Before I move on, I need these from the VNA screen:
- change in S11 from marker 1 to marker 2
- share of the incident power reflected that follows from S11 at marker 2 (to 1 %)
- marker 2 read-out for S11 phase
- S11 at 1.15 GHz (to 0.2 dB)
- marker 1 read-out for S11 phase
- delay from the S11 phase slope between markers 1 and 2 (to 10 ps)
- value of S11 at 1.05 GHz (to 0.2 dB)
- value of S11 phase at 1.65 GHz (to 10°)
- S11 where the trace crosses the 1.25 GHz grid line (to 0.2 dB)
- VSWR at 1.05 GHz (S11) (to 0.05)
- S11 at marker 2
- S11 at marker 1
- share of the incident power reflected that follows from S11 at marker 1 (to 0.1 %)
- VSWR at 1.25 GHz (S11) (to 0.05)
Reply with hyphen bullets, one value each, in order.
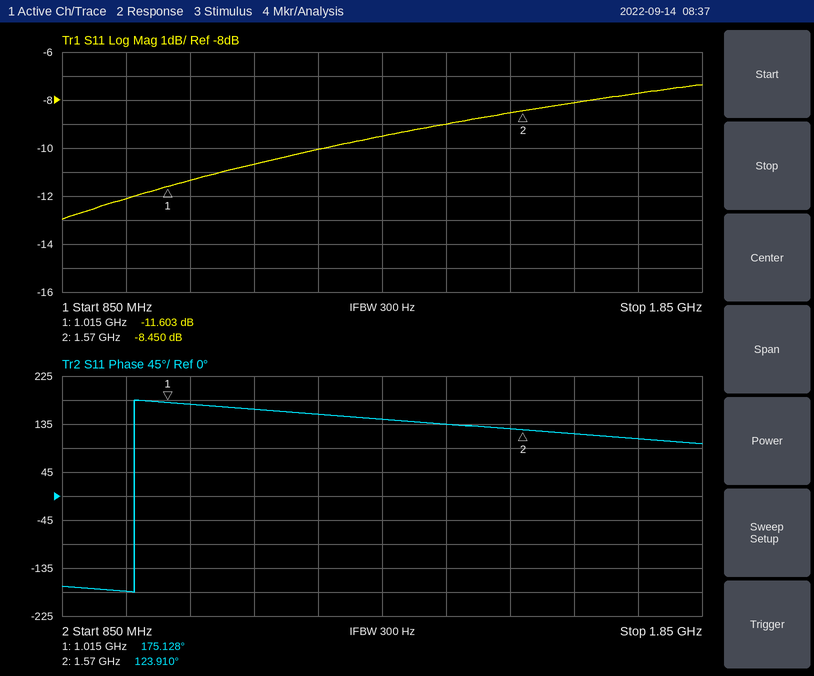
- 3.153 dB
- 14 %
- 123.910°
- -10.6 dB
- 175.128°
- 260 ps
- -11.4 dB
- 120°
- -10.0 dB
- 1.75
- -8.450 dB
- -11.603 dB
- 6.9 %
- 1.90
